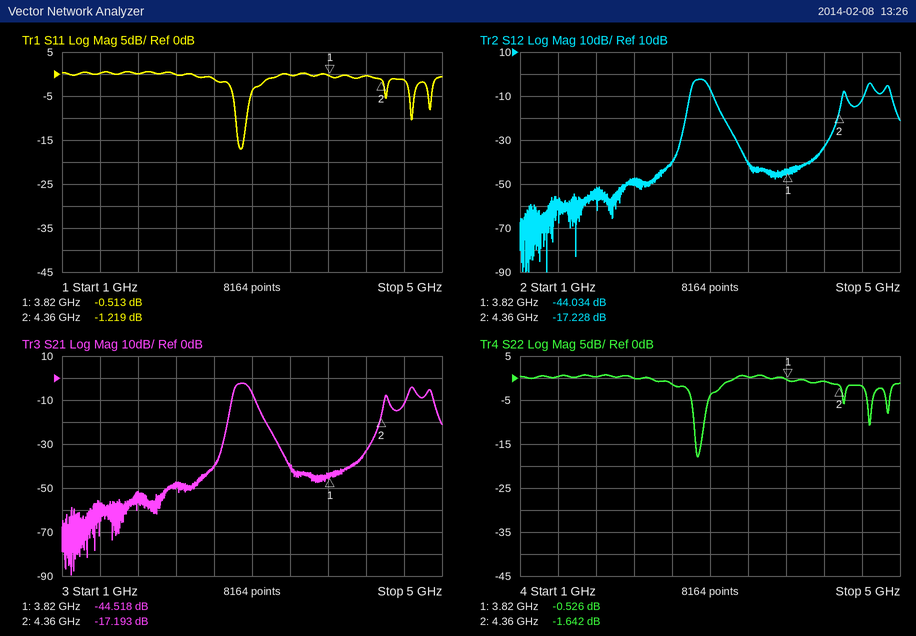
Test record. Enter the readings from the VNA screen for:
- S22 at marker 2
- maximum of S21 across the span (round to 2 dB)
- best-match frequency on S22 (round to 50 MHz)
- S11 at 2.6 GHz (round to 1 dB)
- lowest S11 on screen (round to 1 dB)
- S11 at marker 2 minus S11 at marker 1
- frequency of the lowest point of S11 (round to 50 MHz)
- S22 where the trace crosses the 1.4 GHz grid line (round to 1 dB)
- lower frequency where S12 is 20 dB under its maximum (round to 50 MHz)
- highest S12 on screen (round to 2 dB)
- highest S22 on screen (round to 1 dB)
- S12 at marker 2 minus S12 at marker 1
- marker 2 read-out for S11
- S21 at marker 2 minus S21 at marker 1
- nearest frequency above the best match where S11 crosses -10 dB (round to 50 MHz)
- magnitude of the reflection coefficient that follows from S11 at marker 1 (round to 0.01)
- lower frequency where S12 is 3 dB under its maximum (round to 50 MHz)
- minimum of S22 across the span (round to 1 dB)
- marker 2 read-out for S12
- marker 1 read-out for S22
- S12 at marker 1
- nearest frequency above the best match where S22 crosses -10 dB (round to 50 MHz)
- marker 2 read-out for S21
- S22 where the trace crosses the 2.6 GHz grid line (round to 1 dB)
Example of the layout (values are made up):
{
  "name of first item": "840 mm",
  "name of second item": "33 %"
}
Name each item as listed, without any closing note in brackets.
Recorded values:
{
  "S22 at marker 2": "-1.642 dB",
  "maximum of S21 across the span": "-2 dB",
  "best-match frequency on S22": "2.85 GHz",
  "S11 at 2.6 GHz": "-1 dB",
  "lowest S11 on screen": "-17 dB",
  "S11 at marker 2 minus S11 at marker 1": "-0.706 dB",
  "frequency of the lowest point of S11": "2.90 GHz",
  "S22 where the trace crosses the 1.4 GHz grid line": "0 dB",
  "lower frequency where S12 is 20 dB under its maximum": "2.75 GHz",
  "highest S12 on screen": "-2 dB",
  "highest S22 on screen": "1 dB",
  "S12 at marker 2 minus S12 at marker 1": "26.806 dB",
  "marker 2 read-out for S11": "-1.219 dB",
  "S21 at marker 2 minus S21 at marker 1": "27.325 dB",
  "nearest frequency above the best match where S11 crosses -10 dB": "2.95 GHz",
  "magnitude of the reflection coefficient that follows from S11 at marker 1": "0.94",
  "lower frequency where S12 is 3 dB under its maximum": "2.80 GHz",
  "minimum of S22 across the span": "-18 dB",
  "marker 2 read-out for S12": "-17.228 dB",
  "marker 1 read-out for S22": "-0.526 dB",
  "S12 at marker 1": "-44.034 dB",
  "nearest frequency above the best match where S22 crosses -10 dB": "2.95 GHz",
  "marker 2 read-out for S21": "-17.193 dB",
  "S22 where the trace crosses the 2.6 GHz grid line": "-1 dB"
}
